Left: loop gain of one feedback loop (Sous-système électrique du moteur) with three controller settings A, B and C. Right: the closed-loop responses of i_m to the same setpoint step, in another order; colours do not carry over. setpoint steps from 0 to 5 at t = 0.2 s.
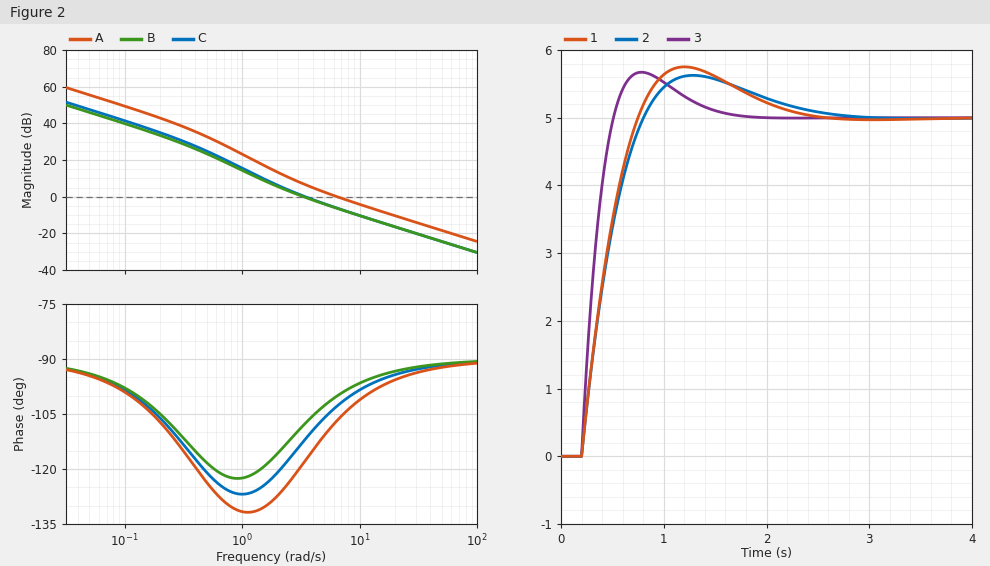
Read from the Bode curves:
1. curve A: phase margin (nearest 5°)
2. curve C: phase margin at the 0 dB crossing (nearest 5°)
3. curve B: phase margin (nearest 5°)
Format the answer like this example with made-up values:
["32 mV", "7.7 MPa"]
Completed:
["75°", "70°", "70°"]
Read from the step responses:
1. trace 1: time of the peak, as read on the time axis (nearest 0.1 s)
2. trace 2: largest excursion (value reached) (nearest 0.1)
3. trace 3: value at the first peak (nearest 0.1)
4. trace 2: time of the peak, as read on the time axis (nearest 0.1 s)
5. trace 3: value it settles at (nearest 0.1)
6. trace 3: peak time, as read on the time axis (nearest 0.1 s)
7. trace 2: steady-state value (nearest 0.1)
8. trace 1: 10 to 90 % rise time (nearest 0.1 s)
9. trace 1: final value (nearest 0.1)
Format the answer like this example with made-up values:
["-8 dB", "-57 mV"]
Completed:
["1.2 s", "5.6", "5.7", "1.3 s", "5.0", "0.8 s", "5.0", "0.4 s", "5.0"]
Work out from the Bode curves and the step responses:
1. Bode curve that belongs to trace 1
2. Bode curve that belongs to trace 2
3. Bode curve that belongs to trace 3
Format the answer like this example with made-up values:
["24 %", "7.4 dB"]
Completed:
["C", "B", "A"]
